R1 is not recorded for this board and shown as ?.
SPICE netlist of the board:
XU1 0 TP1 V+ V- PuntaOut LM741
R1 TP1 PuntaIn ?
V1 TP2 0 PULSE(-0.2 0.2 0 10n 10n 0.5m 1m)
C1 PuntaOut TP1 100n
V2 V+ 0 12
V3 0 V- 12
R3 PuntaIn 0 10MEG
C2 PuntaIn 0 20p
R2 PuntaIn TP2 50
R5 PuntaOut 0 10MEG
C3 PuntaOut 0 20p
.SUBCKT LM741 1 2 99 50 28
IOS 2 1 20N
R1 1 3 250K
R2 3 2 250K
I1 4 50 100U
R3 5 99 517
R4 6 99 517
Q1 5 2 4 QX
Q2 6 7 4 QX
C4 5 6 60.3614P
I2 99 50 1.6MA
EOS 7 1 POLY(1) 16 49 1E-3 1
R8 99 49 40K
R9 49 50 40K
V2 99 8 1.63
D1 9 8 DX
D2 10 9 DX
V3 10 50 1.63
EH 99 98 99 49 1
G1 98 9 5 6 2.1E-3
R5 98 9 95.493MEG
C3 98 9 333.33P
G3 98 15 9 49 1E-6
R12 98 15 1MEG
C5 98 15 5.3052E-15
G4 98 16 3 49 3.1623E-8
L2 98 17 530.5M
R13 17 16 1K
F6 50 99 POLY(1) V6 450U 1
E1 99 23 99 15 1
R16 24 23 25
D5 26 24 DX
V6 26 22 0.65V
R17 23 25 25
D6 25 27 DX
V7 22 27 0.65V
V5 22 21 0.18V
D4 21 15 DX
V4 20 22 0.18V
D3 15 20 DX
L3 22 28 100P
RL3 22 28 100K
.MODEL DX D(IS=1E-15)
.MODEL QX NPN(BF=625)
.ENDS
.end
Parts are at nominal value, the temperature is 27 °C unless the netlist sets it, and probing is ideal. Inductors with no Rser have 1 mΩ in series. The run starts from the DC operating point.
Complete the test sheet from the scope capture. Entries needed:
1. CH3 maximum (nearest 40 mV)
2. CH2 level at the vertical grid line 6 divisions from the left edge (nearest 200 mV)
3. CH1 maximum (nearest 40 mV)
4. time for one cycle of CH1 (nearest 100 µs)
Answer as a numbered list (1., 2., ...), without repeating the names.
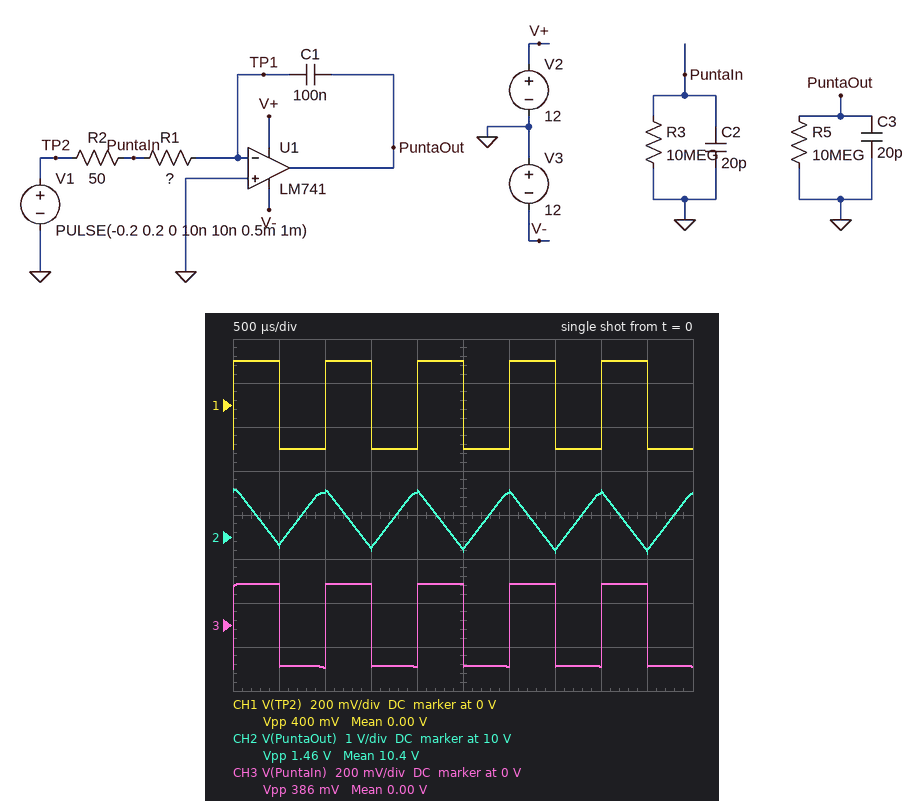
1. 200 mV
2. 11.0 V
3. 200 mV
4. 1.0 ms
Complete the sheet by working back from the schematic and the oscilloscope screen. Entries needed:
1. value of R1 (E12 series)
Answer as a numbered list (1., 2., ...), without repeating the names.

1. 680 Ω
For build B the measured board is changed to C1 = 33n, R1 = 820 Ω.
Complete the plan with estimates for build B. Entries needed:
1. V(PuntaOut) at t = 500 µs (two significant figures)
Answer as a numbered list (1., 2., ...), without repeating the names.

1. 7.7 V
